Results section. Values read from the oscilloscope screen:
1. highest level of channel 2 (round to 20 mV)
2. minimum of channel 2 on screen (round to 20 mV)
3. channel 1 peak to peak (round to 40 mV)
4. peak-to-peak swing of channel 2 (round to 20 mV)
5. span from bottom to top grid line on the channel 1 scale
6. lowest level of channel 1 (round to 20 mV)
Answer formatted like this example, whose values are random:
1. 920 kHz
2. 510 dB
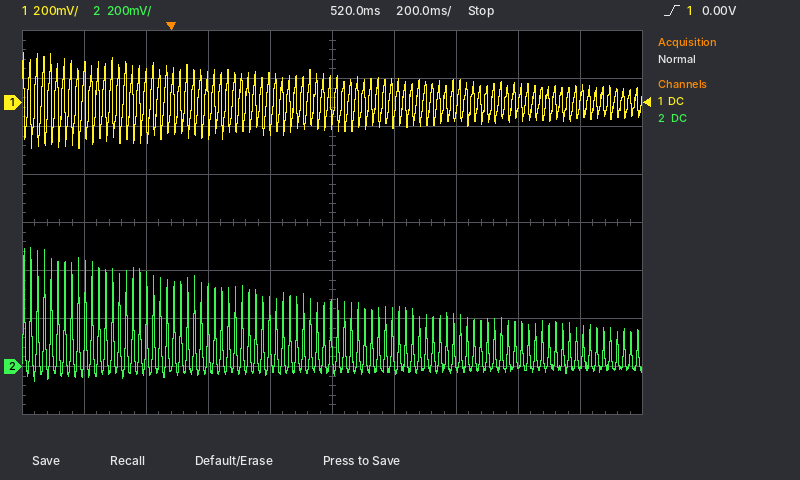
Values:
1. 500 mV
2. -60 mV
3. 400 mV
4. 560 mV
5. 1.6 V
6. -200 mV
